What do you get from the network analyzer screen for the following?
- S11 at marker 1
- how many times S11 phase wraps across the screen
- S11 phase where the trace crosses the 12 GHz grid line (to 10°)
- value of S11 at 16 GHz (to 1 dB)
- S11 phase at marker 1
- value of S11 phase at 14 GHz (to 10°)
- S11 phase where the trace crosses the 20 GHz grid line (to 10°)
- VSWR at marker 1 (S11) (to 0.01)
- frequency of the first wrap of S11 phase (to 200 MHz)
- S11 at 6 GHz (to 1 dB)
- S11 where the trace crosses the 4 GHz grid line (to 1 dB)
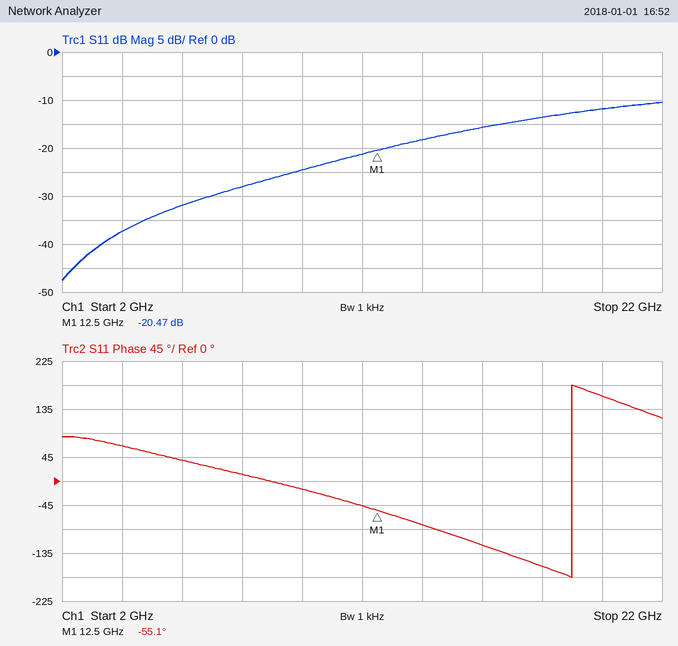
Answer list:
-20.47 dB
1
-50°
-16 dB
-55.1°
-80°
160°
1.21
19.0 GHz
-32 dB
-37 dB
